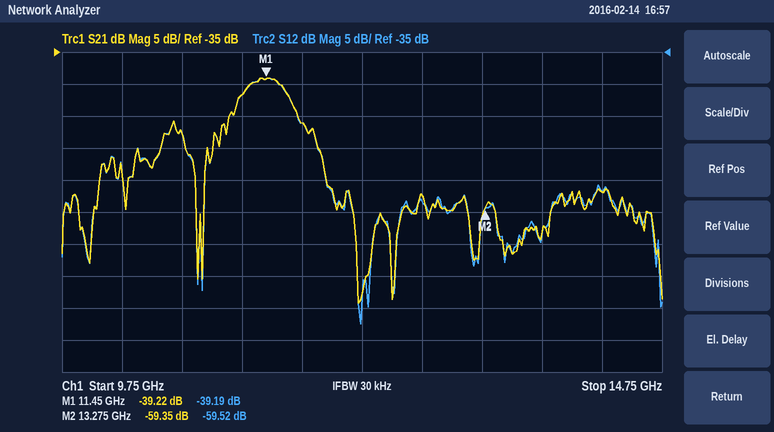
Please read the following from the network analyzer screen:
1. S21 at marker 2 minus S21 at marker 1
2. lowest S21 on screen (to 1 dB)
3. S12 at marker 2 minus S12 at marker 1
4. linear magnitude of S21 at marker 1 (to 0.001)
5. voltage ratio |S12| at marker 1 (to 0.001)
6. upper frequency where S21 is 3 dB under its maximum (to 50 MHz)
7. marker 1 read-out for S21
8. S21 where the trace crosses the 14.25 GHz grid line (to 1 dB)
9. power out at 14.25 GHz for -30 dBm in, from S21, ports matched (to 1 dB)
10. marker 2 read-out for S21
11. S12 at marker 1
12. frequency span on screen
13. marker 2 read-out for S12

-20.13 dB
-74 dB
-20.33 dB
0.011
0.011
11.65 GHz
-39.22 dB
-57 dB
-87 dBm
-59.35 dB
-39.19 dB
5 GHz
-59.52 dB
